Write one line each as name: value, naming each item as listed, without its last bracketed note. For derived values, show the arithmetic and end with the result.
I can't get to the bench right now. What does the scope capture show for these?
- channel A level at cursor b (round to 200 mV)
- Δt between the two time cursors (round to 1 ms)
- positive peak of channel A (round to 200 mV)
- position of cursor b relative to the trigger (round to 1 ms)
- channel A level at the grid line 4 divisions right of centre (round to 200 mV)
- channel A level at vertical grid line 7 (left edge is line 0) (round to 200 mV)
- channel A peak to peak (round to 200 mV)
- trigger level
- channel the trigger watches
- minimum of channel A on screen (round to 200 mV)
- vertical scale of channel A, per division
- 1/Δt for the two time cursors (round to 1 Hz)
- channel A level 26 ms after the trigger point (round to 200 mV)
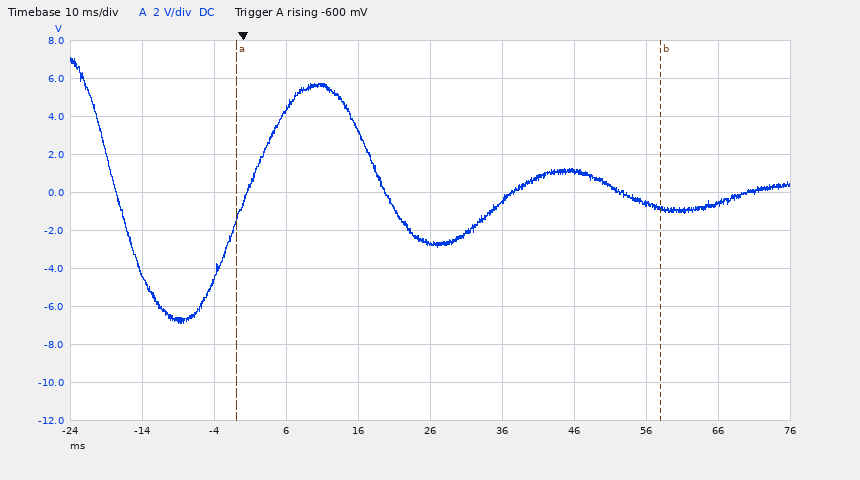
channel A level at cursor b: -800 mV
Δt between the two time cursors: 59 ms
positive peak of channel A: 7.2 V
position of cursor b relative to the trigger: +58 ms
channel A level at the grid line 4 divisions right of centre: -600 mV
channel A level at vertical grid line 7 (left edge is line 0): 1.2 V
channel A peak to peak: 7.2 V − (-6.8 V) = 14.0 V
trigger level: -600 mV
channel the trigger watches: channel A
minimum of channel A on screen: -6.8 V
vertical scale of channel A, per division: 2 V
1/Δt for the two time cursors: 1 / 59 ms ≈ 17 Hz
channel A level 26 ms after the trigger point: -2.6 V
